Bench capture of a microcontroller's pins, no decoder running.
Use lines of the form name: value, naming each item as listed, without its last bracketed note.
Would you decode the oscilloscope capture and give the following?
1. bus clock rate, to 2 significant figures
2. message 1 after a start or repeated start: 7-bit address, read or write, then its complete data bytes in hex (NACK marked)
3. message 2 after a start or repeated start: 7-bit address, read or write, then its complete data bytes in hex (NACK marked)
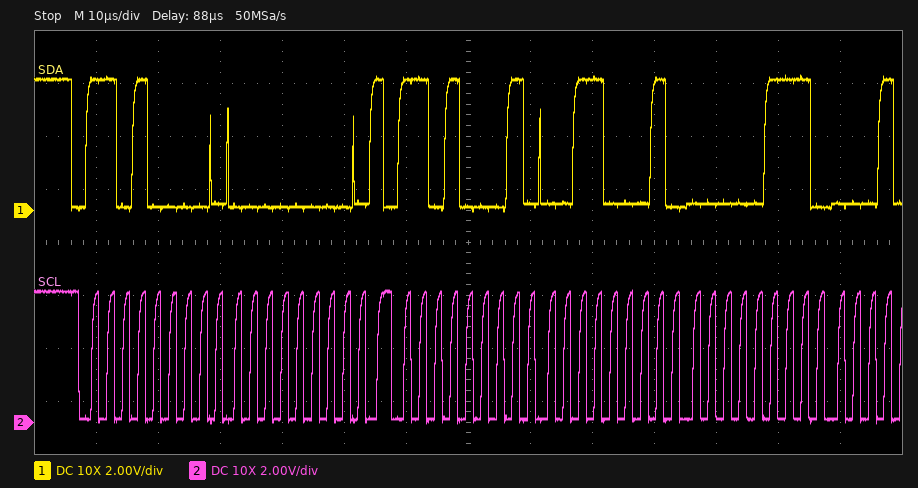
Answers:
bus clock rate, to 2 significant figures: 400 kHz
message 1 after a start or repeated start: 7-bit address, read or write, then its complete data bytes in hex: 0x68 write: 00
message 2 after a start or repeated start: 7-bit address, read or write, then its complete data bytes in hex: 0x68 read: 31 07
